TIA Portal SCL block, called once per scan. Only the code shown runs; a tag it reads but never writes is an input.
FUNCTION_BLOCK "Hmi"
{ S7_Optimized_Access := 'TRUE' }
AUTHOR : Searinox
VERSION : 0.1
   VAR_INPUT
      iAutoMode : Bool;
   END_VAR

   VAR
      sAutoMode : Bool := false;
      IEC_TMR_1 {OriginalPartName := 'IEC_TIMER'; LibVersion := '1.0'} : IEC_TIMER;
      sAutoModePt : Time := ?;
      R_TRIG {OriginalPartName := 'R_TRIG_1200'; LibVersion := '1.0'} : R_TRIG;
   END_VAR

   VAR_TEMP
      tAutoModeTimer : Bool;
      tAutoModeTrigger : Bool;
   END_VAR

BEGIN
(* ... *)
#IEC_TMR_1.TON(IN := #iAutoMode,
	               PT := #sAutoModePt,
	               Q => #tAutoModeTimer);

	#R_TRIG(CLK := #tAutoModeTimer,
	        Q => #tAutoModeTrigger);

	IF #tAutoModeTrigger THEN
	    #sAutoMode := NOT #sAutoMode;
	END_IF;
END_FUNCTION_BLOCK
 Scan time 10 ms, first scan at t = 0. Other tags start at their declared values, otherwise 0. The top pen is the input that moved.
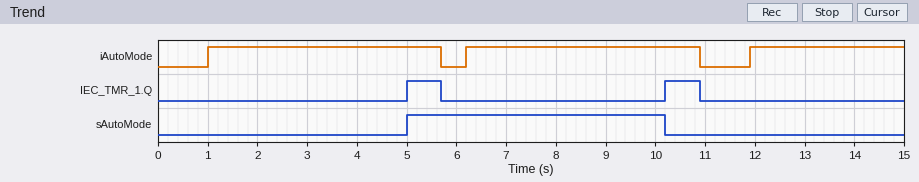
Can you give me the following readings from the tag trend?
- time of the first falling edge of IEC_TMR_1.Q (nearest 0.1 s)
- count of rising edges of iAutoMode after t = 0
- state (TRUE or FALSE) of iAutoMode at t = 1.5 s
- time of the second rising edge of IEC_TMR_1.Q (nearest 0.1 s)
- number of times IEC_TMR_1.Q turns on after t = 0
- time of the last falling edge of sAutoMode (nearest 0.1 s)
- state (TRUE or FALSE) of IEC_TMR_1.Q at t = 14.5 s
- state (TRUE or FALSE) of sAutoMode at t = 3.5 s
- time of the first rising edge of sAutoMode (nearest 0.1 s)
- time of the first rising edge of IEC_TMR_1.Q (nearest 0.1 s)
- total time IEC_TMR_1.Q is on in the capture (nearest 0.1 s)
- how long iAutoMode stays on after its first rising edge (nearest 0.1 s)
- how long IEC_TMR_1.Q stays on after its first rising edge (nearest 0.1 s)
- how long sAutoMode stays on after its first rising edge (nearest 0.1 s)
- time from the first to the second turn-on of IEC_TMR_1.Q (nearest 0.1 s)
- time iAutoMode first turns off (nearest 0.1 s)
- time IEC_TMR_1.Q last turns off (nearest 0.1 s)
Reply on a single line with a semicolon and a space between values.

5.7 s; 3; TRUE; 10.2 s; 2; 10.2 s; FALSE; FALSE; 5.0 s; 5.0 s; 1.4 s; 4.7 s; 0.7 s; 5.2 s; 5.2 s; 5.7 s; 10.9 s
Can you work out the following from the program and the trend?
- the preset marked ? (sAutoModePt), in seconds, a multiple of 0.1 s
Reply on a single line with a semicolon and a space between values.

4.0 s
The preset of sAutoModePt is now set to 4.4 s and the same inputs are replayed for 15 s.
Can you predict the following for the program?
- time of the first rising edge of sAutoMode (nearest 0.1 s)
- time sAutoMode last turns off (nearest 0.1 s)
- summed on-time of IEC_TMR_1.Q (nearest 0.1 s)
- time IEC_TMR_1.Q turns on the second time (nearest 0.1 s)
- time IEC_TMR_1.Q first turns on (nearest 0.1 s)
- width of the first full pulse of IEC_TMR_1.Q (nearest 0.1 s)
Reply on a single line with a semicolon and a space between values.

5.4 s; 10.6 s; 0.6 s; 10.6 s; 5.4 s; 0.3 s
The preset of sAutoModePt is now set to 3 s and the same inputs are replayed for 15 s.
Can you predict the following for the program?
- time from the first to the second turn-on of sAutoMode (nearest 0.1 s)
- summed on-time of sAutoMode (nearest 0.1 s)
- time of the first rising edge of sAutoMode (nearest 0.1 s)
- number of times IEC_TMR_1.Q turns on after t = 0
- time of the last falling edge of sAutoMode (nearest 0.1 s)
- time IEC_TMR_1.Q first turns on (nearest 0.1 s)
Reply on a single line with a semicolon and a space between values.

10.9 s; 5.3 s; 4.0 s; 3; 9.2 s; 4.0 s
